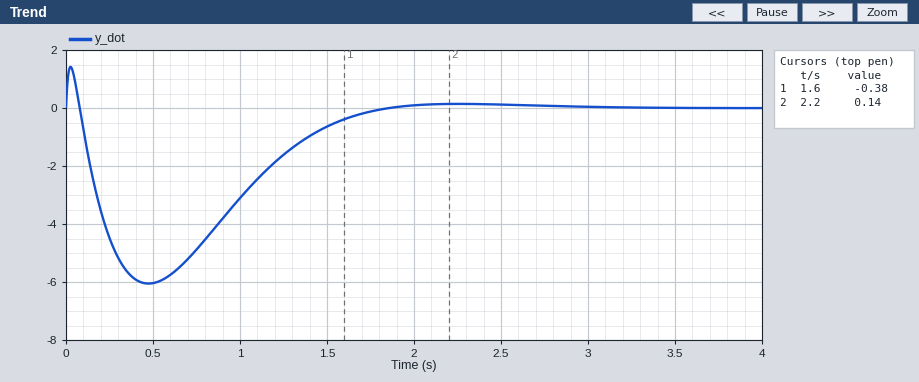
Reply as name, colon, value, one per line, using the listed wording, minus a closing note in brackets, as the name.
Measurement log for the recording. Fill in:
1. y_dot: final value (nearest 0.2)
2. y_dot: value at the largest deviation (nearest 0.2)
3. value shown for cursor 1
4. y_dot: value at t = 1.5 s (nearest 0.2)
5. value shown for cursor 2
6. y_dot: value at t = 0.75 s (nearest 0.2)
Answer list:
y_dot: final value: 0.0
y_dot: value at the largest deviation: -6.0
value shown for cursor 1: -0.38
y_dot: value at t = 1.5 s: -0.6
value shown for cursor 2: 0.14
y_dot: value at t = 0.75 s: -4.8
